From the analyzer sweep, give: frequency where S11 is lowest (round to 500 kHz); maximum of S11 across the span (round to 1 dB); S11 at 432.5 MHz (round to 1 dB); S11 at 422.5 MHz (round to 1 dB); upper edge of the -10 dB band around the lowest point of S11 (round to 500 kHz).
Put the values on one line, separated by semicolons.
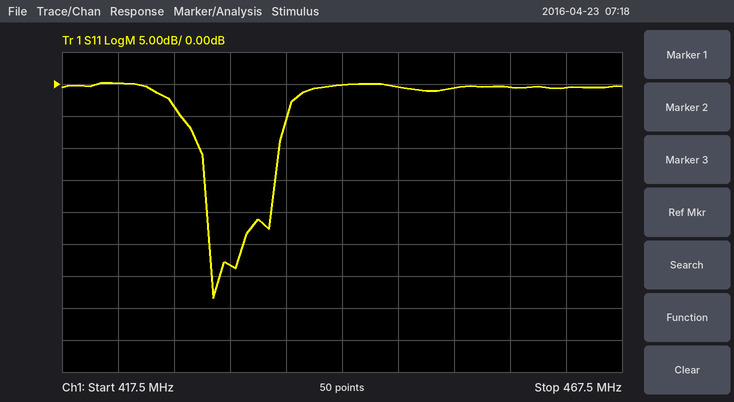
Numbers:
431.0 MHz; 0 dB; -28 dB; 0 dB; 437.0 MHz
